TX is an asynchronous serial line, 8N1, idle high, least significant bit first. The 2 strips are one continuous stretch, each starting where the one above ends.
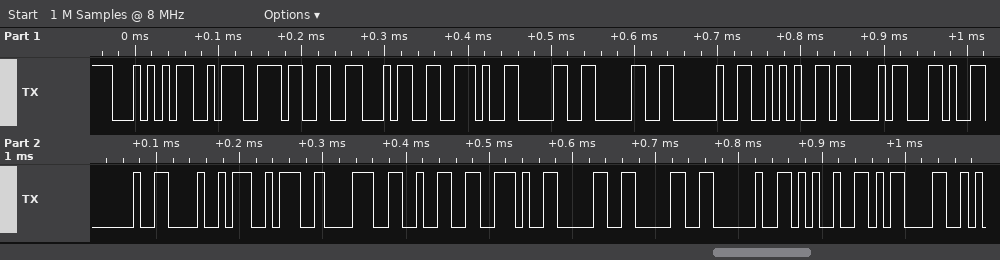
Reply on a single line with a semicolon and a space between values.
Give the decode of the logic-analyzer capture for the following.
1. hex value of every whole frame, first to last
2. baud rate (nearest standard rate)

54 3A 33 34 2E 30 30 20 2A 43 2C 20 48 3A 38 32 2E 30 30 20 25 0D; 115200 baud
